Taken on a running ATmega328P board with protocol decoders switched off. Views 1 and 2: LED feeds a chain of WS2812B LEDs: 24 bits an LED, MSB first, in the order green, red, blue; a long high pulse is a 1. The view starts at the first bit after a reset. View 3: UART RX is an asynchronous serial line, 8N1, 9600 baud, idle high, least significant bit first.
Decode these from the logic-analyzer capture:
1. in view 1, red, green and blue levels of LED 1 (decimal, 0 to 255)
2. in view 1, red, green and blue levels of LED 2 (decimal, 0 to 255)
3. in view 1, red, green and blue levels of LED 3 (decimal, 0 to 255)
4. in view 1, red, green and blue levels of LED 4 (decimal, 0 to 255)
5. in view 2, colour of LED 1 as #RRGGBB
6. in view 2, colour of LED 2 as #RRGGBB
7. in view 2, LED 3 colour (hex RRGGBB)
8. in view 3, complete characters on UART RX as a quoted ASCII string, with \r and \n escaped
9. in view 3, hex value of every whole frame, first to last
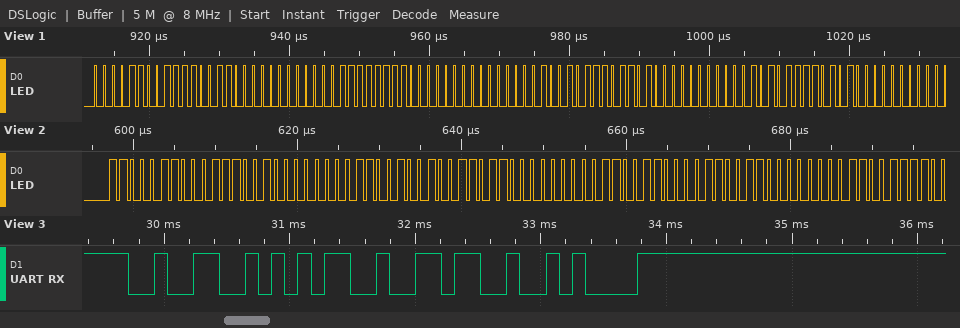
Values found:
243, 12, 0
240, 15, 0
237, 18, 0
234, 21, 0
#39C600
#36C900
#33CC00
"256\n"
32 35 36 0A
